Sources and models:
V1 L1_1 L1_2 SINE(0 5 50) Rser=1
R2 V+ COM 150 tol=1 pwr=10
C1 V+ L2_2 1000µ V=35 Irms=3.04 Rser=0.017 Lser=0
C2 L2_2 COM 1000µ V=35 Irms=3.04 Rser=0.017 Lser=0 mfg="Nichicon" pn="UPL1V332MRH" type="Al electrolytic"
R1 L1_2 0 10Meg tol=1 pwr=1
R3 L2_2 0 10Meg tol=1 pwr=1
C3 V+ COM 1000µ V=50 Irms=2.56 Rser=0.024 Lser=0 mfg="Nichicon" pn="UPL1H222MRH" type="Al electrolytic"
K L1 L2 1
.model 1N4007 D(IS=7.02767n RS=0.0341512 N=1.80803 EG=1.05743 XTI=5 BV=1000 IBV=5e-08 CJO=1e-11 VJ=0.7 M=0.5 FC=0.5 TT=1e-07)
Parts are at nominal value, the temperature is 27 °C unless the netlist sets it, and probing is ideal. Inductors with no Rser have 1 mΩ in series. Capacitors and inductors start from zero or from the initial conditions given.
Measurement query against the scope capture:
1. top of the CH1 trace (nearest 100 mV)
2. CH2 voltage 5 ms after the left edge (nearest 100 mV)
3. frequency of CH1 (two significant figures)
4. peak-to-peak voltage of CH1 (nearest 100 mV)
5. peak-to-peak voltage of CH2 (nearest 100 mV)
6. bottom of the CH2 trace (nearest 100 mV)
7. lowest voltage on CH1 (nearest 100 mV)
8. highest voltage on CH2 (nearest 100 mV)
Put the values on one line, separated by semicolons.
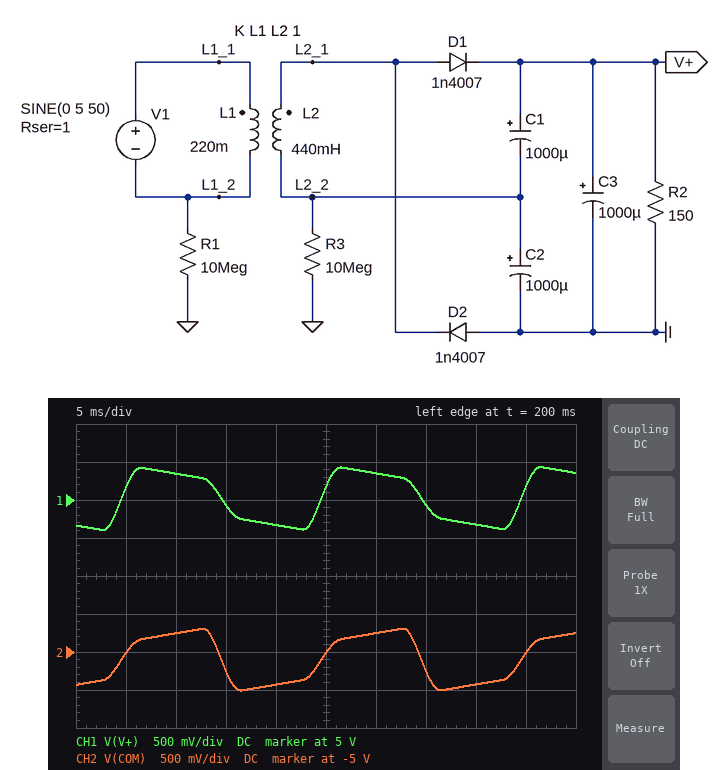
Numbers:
5.4 V; -5.0 V; 50 Hz; 800 mV; 800 mV; -5.5 V; 4.6 V; -4.7 V
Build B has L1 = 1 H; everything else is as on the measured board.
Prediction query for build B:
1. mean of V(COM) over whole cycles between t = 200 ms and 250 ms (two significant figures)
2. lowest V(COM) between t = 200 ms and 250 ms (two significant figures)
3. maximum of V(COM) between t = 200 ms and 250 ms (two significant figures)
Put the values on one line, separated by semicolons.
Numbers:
-2.3 V; -2.5 V; -2.1 V
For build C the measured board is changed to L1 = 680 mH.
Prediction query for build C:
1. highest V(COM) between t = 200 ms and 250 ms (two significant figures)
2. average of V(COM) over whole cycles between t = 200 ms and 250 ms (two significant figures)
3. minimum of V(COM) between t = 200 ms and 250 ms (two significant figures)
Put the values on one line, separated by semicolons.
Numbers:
-2.6 V; -2.9 V; -3.1 V
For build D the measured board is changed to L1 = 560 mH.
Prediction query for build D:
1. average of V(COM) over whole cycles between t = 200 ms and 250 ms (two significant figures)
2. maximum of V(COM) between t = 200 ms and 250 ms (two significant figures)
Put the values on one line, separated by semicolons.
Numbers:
-3.2 V; -2.9 V
